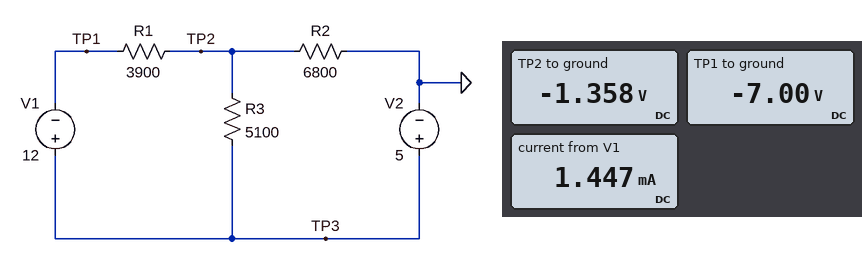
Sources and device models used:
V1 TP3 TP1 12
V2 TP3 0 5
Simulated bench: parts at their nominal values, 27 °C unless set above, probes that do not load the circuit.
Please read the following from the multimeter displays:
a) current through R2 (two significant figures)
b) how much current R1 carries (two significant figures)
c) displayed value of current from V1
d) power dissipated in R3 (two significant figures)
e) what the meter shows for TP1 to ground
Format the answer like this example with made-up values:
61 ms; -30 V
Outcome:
200 µA; 1.4 mA; 1.447 mA; 7.9 mW; -7.00 V
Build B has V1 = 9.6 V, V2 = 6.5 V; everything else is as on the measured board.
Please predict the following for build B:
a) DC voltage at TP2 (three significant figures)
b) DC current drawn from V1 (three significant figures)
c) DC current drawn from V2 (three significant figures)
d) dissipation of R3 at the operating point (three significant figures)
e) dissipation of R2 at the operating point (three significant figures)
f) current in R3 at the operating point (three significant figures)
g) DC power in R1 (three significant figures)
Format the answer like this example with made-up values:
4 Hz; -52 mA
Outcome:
800 mV; 1.00 mA; 118 µA; 6.37 mW; 94.1 µW; 1.12 mA; 3.90 mW
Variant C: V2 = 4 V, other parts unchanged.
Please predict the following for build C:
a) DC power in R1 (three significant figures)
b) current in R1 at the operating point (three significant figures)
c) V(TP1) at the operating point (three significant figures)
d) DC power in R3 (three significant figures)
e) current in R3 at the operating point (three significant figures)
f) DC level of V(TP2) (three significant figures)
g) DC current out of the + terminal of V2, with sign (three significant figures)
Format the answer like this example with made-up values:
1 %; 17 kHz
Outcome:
8.89 mW; 1.51 mA; -8.00 V; 7.33 mW; 1.20 mA; -2.11 V; -311 µA
